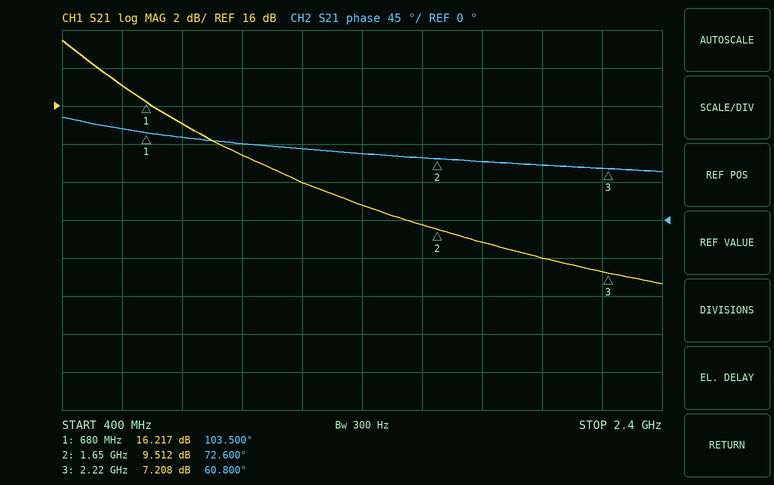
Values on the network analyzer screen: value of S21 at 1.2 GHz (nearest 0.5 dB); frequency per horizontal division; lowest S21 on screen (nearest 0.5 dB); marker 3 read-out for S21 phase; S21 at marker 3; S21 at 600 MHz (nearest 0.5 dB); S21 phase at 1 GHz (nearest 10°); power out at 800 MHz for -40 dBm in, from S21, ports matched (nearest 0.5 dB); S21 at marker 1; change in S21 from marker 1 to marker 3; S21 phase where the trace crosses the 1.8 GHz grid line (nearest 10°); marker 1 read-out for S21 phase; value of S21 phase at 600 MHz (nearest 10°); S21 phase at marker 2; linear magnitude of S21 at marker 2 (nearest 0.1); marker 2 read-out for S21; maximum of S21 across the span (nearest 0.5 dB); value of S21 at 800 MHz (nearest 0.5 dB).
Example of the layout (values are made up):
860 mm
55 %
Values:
12.0 dB
200 MHz
6.5 dB
60.800°
7.208 dB
17.0 dB
90°
-25.0 dBm
16.217 dB
-9.009 dB
70°
103.500°
110°
72.600°
3.0
9.512 dB
19.5 dB
15.0 dB
